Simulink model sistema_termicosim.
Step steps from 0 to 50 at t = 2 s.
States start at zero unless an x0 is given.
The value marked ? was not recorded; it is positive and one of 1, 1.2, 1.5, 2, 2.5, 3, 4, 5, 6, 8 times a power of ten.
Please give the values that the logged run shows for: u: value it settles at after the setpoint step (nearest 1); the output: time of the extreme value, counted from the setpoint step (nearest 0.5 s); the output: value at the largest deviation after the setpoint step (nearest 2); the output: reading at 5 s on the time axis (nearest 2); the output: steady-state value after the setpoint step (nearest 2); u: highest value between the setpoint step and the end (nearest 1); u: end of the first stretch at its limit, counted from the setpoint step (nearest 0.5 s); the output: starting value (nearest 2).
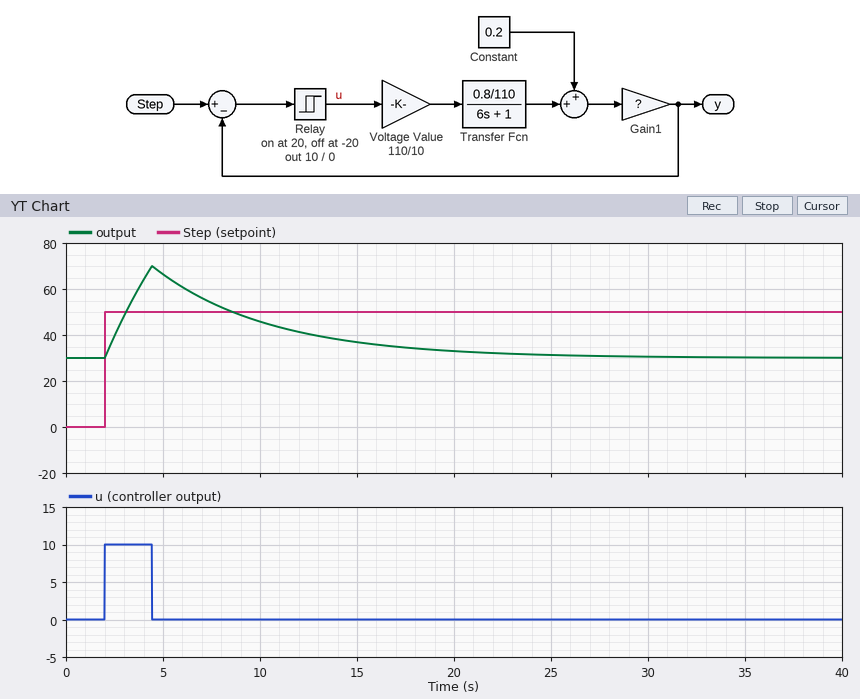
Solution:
0
2.5 s
70
66
30
10
2.5 s
30
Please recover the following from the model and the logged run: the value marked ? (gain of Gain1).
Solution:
150
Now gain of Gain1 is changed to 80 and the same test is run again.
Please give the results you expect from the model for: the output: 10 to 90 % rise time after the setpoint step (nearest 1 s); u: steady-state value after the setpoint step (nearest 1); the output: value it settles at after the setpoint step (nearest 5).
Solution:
8 s
10
70
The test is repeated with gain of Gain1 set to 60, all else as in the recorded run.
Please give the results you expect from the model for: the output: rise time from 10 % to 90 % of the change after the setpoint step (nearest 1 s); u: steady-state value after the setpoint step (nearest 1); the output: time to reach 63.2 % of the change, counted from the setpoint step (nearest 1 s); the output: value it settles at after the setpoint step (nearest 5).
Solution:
13 s
10
6 s
60
